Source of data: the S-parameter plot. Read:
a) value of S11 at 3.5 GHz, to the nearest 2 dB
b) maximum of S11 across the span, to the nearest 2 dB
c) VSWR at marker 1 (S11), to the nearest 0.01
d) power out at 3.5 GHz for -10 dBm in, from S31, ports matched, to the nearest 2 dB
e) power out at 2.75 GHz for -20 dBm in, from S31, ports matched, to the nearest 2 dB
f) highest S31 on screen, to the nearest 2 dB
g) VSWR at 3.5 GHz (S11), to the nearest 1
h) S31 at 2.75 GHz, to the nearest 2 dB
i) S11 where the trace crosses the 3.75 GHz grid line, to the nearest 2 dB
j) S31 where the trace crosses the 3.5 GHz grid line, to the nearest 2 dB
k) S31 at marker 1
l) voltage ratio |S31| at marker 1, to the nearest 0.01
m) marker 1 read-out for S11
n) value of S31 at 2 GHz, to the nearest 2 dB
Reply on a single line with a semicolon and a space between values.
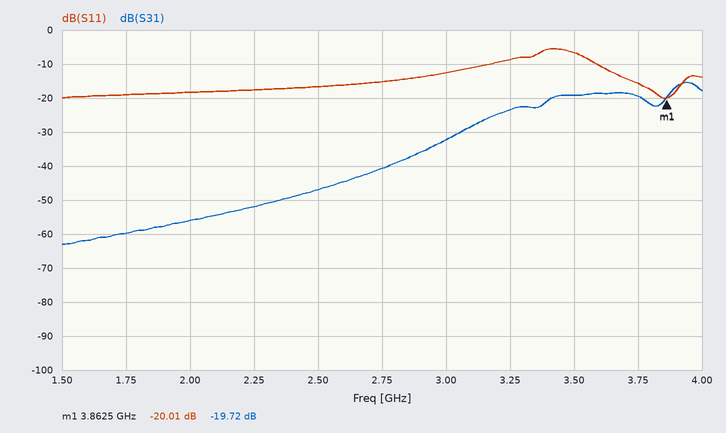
-6 dB; -6 dB; 1.22; -30 dBm; -60 dBm; -16 dB; 3; -40 dB; -16 dB; -20 dB; -19.72 dB; 0.10; -20.01 dB; -56 dB
